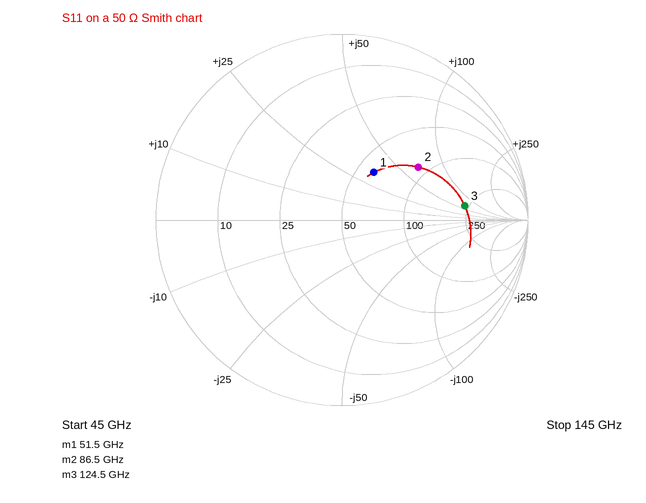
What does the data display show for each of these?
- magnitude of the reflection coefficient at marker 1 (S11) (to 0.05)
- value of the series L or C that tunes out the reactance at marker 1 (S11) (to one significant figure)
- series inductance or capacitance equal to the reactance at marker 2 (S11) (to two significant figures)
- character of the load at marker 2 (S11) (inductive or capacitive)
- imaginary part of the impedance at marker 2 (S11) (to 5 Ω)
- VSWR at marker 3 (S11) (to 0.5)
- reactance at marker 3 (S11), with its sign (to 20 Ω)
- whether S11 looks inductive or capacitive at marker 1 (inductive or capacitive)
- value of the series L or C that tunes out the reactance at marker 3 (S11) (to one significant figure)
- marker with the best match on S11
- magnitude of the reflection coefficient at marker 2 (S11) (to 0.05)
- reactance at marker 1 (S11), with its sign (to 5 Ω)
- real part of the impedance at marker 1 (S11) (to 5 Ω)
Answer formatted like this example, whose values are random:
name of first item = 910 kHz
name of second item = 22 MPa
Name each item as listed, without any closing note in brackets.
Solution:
magnitude of the reflection coefficient at marker 1 (S11) = 0.30
value of the series L or C that tunes out the reactance at marker 1 (S11) = 90 fF
series inductance or capacitance equal to the reactance at marker 2 (S11) = 120 pH
character of the load at marker 2 (S11) = inductive
imaginary part of the impedance at marker 2 (S11) = +65 Ω
VSWR at marker 3 (S11) = 5.0
reactance at marker 3 (S11), with its sign = +60 Ω
whether S11 looks inductive or capacitive at marker 1 = inductive
value of the series L or C that tunes out the reactance at marker 3 (S11) = 20 fF
marker with the best match on S11 = marker 1
magnitude of the reflection coefficient at marker 2 (S11) = 0.50
reactance at marker 1 (S11), with its sign = +35 Ω
real part of the impedance at marker 1 (S11) = 60 Ω
